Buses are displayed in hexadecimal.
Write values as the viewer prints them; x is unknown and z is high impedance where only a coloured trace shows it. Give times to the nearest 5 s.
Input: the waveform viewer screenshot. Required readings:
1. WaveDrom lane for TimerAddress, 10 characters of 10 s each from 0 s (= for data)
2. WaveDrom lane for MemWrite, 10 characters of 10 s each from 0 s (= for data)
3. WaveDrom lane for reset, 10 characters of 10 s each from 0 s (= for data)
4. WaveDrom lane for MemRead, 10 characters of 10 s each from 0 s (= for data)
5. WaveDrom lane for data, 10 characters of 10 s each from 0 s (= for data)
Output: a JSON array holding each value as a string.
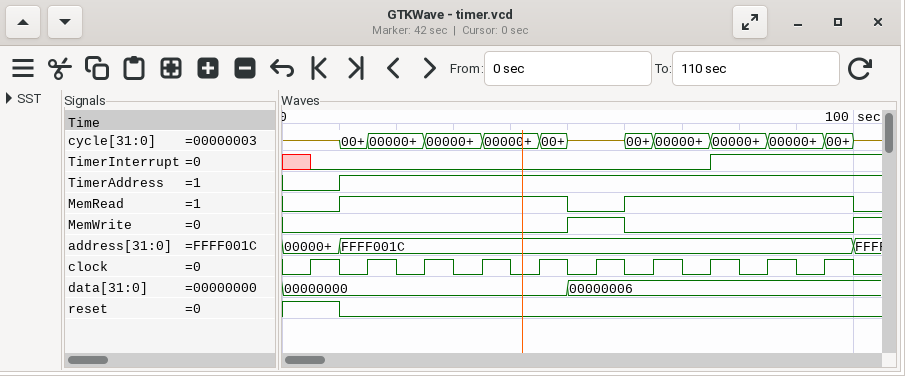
["{name: 'TimerAddress', wave: '01........'}", "{name: 'MemWrite', wave: '0....10...'}", "{name: 'reset', wave: '10........'}", "{name: 'MemRead', wave: '01...01...'}", "{name: 'data', wave: '=....=....', data: '00000000 00000006'}"]
